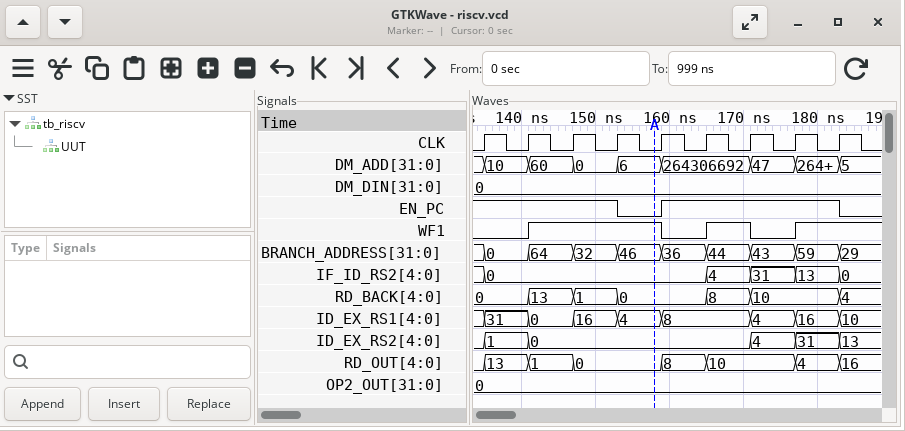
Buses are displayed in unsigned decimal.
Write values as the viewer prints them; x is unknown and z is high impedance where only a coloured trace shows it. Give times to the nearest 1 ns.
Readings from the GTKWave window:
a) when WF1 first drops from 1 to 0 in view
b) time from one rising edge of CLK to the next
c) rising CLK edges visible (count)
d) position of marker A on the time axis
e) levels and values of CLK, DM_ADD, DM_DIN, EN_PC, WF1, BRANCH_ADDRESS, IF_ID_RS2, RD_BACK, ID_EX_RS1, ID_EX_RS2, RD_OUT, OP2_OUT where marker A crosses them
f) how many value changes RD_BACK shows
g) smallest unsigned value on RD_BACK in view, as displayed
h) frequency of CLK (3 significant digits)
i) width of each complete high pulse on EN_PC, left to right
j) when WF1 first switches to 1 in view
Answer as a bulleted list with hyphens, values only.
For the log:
- 159 ns
- 6 ns
- 9
- 158 ns
- CLK=0, DM_ADD=6, DM_DIN=0, EN_PC=0, WF1=1, BRANCH_ADDRESS=46, IF_ID_RS2=0, RD_BACK=0, ID_EX_RS1=4, ID_EX_RS2=0, RD_OUT=0, OP2_OUT=0
- 6
- 0
- 167 MHz
- 24 ns
- 141 ns
